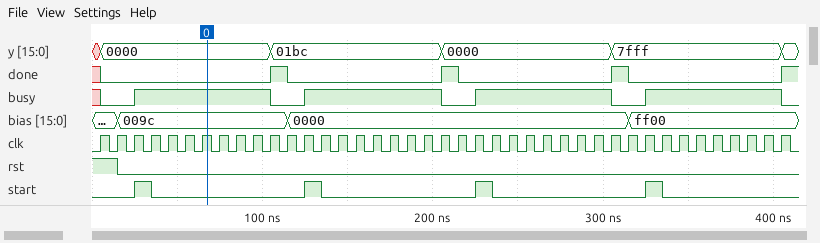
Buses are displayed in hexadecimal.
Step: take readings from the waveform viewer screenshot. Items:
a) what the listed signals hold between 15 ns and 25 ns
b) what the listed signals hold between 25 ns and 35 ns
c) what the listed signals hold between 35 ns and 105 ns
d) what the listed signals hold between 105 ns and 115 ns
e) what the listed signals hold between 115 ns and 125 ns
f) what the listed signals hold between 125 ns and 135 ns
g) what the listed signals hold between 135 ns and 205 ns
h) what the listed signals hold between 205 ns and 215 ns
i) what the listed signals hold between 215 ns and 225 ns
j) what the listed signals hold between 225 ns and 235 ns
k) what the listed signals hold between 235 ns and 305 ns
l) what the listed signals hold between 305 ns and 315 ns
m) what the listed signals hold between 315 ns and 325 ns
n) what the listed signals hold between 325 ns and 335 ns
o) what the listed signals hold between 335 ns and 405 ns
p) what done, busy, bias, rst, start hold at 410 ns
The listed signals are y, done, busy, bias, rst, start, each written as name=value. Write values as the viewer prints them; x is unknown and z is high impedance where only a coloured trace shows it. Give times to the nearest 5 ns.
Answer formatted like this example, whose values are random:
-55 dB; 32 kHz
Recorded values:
y=0000, done=0, busy=0, bias=009c, rst=0, start=0; y=0000, done=0, busy=1, bias=009c, rst=0, start=1; y=0000, done=0, busy=1, bias=009c, rst=0, start=0; y=01bc, done=1, busy=0, bias=009c, rst=0, start=0; y=01bc, done=0, busy=0, bias=0000, rst=0, start=0; y=01bc, done=0, busy=1, bias=0000, rst=0, start=1; y=01bc, done=0, busy=1, bias=0000, rst=0, start=0; y=0000, done=1, busy=0, bias=0000, rst=0, start=0; y=0000, done=0, busy=0, bias=0000, rst=0, start=0; y=0000, done=0, busy=1, bias=0000, rst=0, start=1; y=0000, done=0, busy=1, bias=0000, rst=0, start=0; y=7fff, done=1, busy=0, bias=0000, rst=0, start=0; y=7fff, done=0, busy=0, bias=ff00, rst=0, start=0; y=7fff, done=0, busy=1, bias=ff00, rst=0, start=1; y=7fff, done=0, busy=1, bias=ff00, rst=0, start=0; done=1, busy=0, bias=ff00, rst=0, start=0
